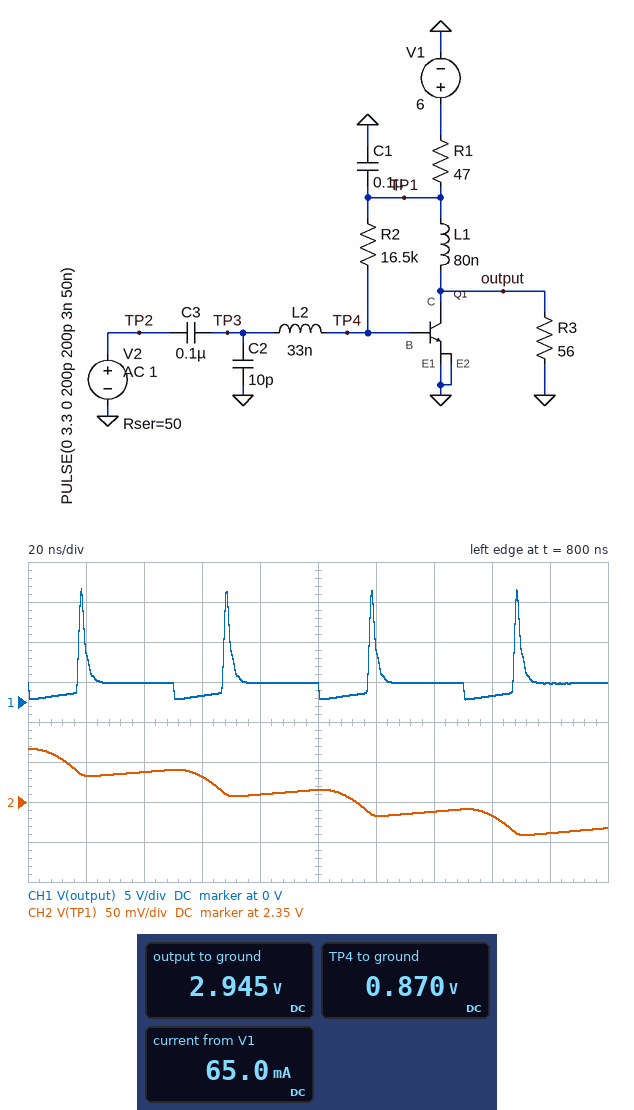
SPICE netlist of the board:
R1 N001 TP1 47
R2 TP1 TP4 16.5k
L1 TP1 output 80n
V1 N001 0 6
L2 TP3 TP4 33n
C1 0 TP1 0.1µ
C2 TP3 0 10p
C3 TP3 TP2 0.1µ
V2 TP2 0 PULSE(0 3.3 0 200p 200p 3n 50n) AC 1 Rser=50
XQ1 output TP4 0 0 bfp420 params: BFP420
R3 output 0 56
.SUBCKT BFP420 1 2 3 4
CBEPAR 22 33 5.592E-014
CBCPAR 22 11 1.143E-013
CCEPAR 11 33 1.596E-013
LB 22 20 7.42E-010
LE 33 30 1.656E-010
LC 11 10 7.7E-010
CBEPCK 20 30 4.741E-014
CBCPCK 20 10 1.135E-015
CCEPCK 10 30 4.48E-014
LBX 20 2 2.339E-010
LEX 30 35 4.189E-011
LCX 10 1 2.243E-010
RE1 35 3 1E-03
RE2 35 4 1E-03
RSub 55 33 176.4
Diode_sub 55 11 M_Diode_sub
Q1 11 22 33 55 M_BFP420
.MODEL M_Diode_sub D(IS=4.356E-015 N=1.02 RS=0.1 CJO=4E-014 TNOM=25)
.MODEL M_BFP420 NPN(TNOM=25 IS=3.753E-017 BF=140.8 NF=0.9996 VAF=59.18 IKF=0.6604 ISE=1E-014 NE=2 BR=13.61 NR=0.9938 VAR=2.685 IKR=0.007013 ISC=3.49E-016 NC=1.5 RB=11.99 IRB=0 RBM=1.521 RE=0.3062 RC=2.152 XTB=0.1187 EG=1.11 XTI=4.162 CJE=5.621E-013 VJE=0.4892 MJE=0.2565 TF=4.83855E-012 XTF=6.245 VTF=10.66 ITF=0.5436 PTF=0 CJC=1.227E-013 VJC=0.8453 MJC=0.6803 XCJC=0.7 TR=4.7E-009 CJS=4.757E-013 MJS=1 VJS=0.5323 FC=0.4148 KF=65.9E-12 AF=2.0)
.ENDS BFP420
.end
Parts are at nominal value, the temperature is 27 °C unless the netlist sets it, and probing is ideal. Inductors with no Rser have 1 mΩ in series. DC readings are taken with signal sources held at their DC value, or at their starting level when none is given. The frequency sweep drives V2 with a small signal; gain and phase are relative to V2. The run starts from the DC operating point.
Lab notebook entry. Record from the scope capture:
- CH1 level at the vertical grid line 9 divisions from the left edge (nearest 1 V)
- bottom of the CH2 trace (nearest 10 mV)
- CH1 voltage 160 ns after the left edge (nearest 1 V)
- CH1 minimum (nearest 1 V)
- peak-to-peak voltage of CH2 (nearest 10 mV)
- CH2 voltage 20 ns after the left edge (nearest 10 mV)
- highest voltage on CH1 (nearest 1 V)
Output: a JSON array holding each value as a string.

["2 V", "2.31 V", "1 V", "0 V", "110 mV", "2.38 V", "14 V"]
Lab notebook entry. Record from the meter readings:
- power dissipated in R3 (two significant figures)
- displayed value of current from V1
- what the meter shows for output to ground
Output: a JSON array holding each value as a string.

["150 mW", "65.0 mA", "2.945 V"]
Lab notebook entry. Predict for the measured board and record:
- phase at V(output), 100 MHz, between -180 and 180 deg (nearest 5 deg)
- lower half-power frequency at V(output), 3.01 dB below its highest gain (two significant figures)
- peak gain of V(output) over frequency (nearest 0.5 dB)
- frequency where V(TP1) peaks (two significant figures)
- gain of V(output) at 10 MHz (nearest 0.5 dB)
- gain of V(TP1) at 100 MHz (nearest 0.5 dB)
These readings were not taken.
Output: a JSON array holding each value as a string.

["-160 deg", "120 MHz", "25.5 dB", "20 kHz", "4.0 dB", "-48.5 dB"]
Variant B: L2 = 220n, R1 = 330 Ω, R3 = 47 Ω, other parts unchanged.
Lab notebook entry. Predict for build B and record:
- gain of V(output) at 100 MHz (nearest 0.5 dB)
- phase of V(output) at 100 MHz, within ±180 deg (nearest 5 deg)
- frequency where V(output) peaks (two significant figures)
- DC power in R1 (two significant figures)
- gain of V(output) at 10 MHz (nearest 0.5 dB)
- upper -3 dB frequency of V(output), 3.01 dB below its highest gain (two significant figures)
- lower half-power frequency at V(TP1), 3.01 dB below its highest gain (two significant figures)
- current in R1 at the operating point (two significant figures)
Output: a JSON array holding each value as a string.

["-19.5 dB", "-160 deg", "300 MHz", "84 mW", "-37.0 dB", "320 MHz", "150 Hz", "16 mA"]
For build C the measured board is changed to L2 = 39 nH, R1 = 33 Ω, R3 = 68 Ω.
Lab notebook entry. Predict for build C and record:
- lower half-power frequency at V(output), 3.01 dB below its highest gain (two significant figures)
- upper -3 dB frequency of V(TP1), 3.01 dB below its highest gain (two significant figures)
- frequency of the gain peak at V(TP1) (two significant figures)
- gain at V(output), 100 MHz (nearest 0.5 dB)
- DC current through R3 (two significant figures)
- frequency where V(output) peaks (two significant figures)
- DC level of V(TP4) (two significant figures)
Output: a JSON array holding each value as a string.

["140 MHz", "87 kHz", "23 kHz", "24.0 dB", "54 mA", "300 MHz", "880 mV"]
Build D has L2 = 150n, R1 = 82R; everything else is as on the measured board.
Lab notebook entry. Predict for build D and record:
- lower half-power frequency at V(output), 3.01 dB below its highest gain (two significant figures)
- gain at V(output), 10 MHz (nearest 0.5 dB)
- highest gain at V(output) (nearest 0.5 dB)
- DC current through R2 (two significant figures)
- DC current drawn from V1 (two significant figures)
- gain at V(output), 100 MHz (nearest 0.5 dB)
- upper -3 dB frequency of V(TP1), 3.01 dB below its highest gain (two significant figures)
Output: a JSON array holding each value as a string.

["140 MHz", "1.0 dB", "26.0 dB", "80 µA", "47 mA", "20.0 dB", "57 kHz"]
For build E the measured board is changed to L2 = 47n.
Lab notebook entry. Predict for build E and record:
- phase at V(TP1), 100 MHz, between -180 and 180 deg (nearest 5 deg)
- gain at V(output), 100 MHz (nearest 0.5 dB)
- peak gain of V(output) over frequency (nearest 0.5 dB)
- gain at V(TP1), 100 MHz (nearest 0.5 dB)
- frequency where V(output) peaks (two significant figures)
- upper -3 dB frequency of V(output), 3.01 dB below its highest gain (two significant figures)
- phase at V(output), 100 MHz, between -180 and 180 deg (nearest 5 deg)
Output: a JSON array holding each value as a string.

["15 deg", "22.0 dB", "26.5 dB", "-48.0 dB", "310 MHz", "390 MHz", "-165 deg"]
